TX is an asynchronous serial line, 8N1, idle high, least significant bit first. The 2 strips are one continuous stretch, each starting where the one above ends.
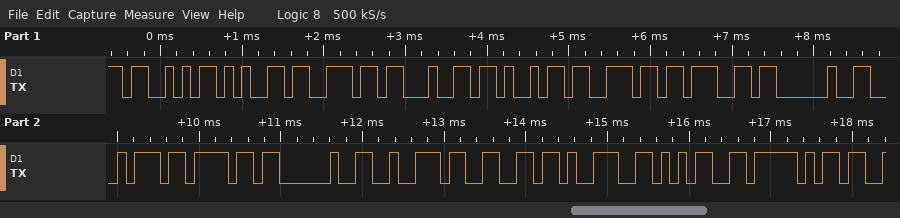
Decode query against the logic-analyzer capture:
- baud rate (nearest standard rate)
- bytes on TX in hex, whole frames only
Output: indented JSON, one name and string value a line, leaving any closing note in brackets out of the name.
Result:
{
  "baud rate": "9600 baud",
  "bytes on TX in hex, whole frames only": "0x53 0x65 0x6E 0x64 0x69 0x6E 0x67 0x20 0x74 0x6F 0x20 0x72 0x66 0x39 0x35 0x5F"
}
